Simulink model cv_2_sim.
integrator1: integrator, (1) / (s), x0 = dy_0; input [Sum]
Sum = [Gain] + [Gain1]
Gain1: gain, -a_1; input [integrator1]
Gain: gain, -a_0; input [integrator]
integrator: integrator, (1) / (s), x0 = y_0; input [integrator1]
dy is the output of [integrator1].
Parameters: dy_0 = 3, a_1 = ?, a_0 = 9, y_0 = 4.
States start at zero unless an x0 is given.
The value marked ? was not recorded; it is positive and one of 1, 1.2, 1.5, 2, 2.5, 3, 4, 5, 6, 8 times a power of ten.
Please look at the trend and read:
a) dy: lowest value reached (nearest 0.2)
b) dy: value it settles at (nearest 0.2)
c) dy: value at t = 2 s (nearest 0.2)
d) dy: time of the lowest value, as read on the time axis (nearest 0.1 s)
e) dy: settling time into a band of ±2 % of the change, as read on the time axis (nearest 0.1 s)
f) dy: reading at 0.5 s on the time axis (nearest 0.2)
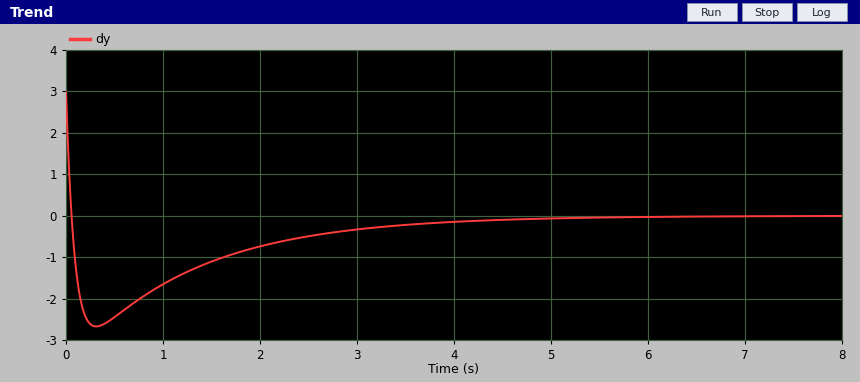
-2.6
0.0
-0.8
0.3 s
5.1 s
-2.4
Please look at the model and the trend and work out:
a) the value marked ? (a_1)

12
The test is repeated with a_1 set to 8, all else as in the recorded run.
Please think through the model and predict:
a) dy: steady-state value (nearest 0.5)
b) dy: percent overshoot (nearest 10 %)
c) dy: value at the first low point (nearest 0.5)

0.0
120 %
-3.5
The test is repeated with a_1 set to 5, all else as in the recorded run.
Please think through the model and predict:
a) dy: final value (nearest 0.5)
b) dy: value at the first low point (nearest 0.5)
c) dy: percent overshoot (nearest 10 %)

0.0
-5.0
170 %
